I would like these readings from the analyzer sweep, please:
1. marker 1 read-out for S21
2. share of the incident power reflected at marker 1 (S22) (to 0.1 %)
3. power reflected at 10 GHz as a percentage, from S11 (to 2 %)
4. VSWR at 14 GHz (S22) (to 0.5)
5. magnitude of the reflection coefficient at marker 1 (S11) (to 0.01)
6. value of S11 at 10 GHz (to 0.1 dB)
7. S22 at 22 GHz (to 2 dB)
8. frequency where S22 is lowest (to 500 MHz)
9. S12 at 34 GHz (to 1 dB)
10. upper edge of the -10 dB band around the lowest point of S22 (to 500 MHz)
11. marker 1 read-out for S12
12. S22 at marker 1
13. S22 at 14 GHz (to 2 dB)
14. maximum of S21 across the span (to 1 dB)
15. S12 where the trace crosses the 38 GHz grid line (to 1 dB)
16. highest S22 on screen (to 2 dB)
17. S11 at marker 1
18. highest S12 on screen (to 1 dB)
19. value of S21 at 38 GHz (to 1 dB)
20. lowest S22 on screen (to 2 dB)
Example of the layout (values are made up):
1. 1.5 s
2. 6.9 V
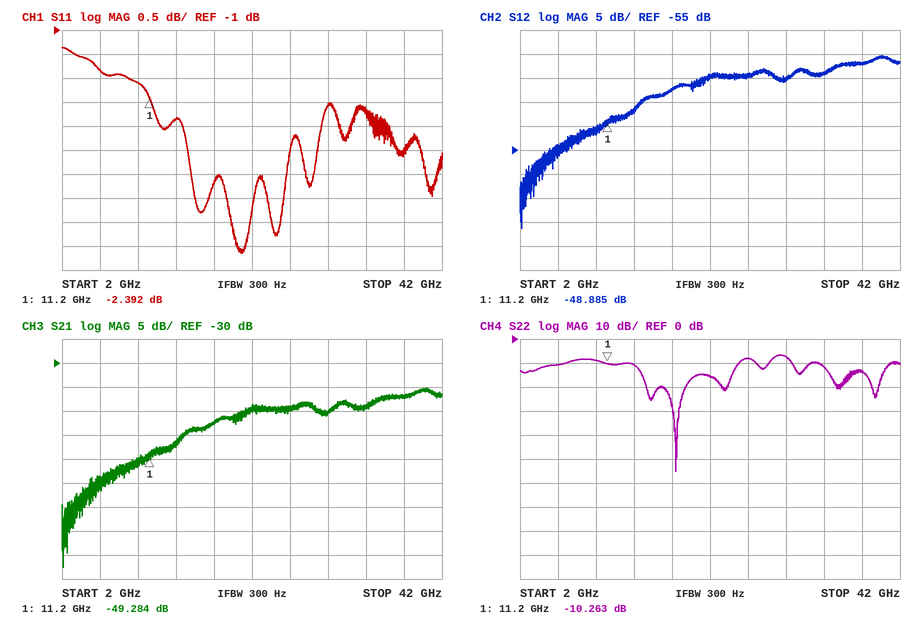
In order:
1. -49.284 dB
2. 9.4 %
3. 62 %
4. 2.0
5. 0.76
6. -2.1 dB
7. -16 dB
8. 18.5 GHz
9. -39 dB
10. 25.0 GHz
11. -48.885 dB
12. -10.263 dB
13. -10 dB
14. -35 dB
15. -37 dB
16. -6 dB
17. -2.392 dB
18. -35 dB
19. -37 dB
20. -56 dB
